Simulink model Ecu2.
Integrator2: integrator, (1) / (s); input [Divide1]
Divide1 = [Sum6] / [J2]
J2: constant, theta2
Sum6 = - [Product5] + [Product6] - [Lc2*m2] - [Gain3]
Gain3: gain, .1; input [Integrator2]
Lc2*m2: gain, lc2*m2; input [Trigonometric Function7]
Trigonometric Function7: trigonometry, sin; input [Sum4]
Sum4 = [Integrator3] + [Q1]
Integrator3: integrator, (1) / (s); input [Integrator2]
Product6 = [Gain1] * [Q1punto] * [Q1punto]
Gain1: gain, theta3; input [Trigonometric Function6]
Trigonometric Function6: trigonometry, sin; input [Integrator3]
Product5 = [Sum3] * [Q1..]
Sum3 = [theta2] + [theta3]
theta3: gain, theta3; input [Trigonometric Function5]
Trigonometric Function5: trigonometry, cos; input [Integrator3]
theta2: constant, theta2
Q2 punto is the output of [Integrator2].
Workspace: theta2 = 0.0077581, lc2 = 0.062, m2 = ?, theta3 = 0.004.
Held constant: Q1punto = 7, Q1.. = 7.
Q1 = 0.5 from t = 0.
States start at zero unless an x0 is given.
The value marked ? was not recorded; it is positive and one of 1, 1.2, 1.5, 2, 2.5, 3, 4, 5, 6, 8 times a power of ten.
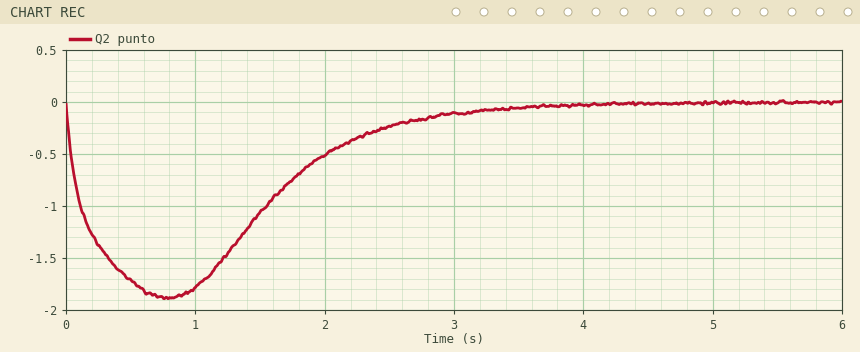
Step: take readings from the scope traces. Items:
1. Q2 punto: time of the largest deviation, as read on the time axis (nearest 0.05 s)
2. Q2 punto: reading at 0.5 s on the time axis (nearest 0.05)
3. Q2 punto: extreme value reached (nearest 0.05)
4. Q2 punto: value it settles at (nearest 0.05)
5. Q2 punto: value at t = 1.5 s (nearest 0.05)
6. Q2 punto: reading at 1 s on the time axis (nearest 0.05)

0.80 s
-1.70
-1.90
0.00
-1.05
-1.80
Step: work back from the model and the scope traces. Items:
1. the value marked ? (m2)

1.5
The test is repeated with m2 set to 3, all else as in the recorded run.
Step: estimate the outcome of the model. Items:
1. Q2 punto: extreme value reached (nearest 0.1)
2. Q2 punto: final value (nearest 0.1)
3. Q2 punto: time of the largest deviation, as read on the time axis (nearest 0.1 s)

-1.7
0.0
0.4 s
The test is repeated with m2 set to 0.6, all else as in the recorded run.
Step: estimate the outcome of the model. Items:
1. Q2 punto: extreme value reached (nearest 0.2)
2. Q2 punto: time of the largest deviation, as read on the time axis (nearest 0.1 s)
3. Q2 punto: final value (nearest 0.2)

-2.2
1.0 s
0.0
